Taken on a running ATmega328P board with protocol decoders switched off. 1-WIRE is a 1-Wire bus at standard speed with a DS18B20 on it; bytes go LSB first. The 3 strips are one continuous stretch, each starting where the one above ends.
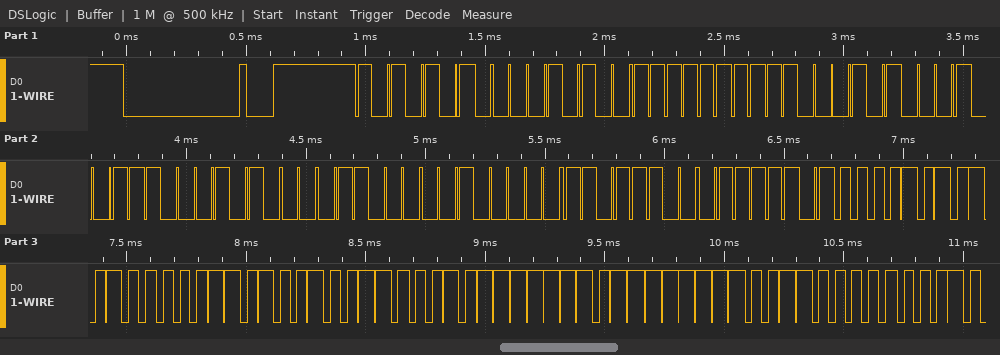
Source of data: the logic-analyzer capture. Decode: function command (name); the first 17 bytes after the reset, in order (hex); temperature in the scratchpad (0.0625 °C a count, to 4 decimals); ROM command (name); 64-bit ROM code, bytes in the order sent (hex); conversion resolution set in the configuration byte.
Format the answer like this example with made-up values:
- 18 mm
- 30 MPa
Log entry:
- Read Scratchpad
- 55 28 FF A3 C8 51 18 04 3B BE 50 05 4B 46 7F FF 0C
- 85.0000 °C
- Match ROM
- 28 FF A3 C8 51 18 04 3B
- 12 bits
